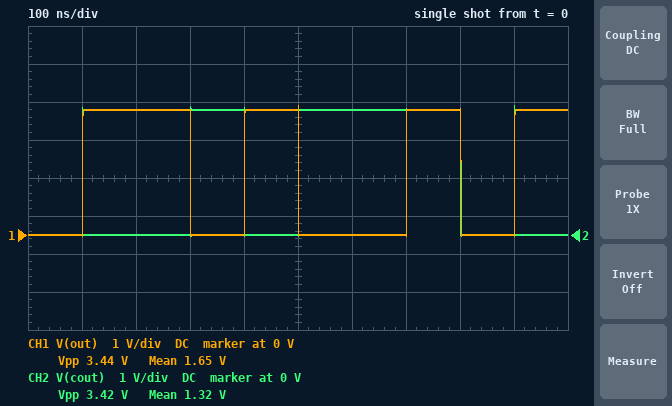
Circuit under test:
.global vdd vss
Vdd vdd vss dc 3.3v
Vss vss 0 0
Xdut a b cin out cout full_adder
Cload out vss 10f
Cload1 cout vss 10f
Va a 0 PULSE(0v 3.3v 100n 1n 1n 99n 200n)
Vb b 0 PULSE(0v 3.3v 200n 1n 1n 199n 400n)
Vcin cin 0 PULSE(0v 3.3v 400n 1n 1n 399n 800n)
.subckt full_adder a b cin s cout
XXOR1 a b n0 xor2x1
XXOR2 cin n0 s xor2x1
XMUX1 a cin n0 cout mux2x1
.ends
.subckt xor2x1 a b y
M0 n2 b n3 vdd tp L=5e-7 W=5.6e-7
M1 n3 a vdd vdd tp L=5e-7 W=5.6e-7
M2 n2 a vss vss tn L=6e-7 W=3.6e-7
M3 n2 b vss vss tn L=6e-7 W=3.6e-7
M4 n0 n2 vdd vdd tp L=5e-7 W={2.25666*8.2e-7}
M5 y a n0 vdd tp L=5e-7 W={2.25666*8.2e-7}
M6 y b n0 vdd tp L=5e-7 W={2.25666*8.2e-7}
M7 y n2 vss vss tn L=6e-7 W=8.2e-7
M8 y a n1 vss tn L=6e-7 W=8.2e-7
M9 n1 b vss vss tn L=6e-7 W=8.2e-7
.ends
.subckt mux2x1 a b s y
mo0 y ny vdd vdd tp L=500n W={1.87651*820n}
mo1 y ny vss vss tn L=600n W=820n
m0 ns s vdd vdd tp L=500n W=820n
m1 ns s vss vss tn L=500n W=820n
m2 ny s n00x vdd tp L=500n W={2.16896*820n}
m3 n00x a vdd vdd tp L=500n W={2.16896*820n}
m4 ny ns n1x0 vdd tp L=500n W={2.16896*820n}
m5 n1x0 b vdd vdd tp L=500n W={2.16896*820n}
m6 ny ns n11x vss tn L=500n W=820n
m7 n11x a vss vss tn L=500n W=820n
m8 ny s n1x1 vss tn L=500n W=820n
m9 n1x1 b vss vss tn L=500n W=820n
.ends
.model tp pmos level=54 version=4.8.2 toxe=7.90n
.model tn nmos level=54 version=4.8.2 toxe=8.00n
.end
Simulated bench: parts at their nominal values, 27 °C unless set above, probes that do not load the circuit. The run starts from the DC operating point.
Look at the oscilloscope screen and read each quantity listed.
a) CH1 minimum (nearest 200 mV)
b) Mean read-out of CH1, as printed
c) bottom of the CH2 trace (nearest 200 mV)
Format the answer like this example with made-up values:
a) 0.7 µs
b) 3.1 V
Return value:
a) 0 V
b) 1.65 V
c) 0 V
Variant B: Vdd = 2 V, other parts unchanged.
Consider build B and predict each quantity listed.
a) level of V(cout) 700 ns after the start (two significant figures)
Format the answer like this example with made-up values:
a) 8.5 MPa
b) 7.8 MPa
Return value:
a) 2.0 V
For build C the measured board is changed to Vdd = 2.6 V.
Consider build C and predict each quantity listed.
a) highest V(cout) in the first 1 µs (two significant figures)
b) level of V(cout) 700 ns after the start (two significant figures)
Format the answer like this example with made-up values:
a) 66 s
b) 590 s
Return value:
a) 2.7 V
b) 2.6 V
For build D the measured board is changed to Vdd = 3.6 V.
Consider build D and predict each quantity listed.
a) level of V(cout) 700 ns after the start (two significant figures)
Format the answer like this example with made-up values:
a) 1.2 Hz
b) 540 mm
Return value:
a) 3.6 V
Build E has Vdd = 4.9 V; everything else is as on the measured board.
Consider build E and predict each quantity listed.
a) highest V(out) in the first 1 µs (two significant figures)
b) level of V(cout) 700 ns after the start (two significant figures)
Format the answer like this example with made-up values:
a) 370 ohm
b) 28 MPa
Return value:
a) 5.0 V
b) 4.9 V
